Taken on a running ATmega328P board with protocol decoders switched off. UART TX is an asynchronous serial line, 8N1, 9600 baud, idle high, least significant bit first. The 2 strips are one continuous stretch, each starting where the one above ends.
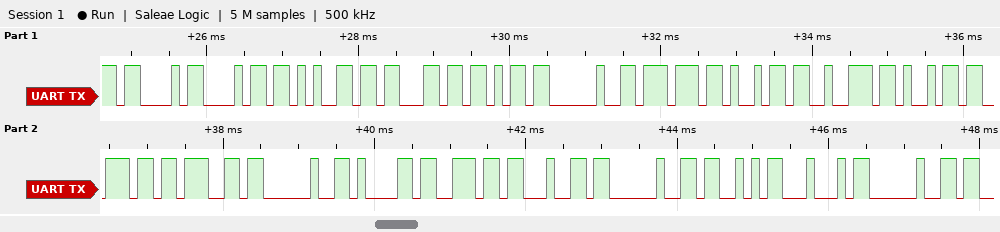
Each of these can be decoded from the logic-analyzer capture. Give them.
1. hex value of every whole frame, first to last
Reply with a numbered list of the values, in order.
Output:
1. 0x43 0x68 0x65 0x63 0x6B 0x20 0x77 0x69 0x72 0x69 0x6E 0x67 0x20 0x61 0x6E 0x64 0x20 0x53 0x44 0x20
